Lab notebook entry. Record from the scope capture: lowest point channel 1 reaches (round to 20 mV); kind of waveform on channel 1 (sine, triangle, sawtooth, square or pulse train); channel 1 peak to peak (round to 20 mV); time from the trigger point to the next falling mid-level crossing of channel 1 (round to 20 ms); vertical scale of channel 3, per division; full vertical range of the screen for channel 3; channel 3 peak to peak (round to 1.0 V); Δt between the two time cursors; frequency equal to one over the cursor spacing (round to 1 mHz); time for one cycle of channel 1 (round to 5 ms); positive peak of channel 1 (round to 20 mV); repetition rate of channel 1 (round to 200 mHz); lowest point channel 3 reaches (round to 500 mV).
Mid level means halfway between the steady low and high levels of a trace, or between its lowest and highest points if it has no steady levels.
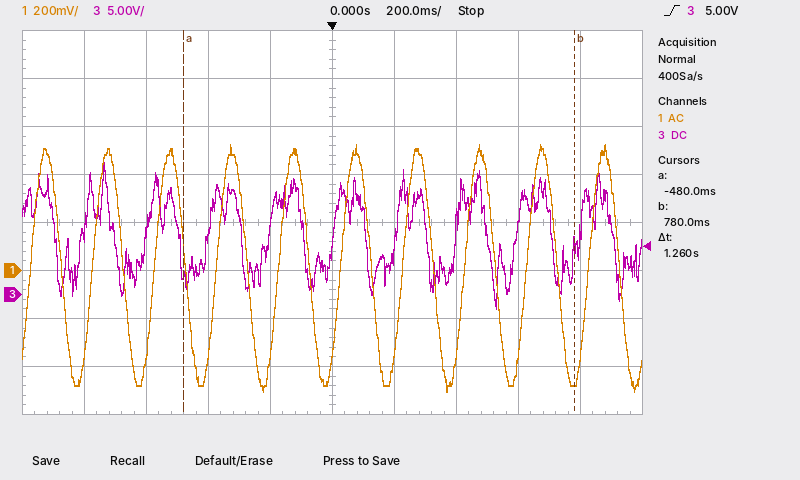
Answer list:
-500 mV
sine
1.02 V
120 ms
5 V
40 V
15.0 V
1.26 s
794 mHz
200 ms
520 mV
5.0 Hz
-1.5 V
